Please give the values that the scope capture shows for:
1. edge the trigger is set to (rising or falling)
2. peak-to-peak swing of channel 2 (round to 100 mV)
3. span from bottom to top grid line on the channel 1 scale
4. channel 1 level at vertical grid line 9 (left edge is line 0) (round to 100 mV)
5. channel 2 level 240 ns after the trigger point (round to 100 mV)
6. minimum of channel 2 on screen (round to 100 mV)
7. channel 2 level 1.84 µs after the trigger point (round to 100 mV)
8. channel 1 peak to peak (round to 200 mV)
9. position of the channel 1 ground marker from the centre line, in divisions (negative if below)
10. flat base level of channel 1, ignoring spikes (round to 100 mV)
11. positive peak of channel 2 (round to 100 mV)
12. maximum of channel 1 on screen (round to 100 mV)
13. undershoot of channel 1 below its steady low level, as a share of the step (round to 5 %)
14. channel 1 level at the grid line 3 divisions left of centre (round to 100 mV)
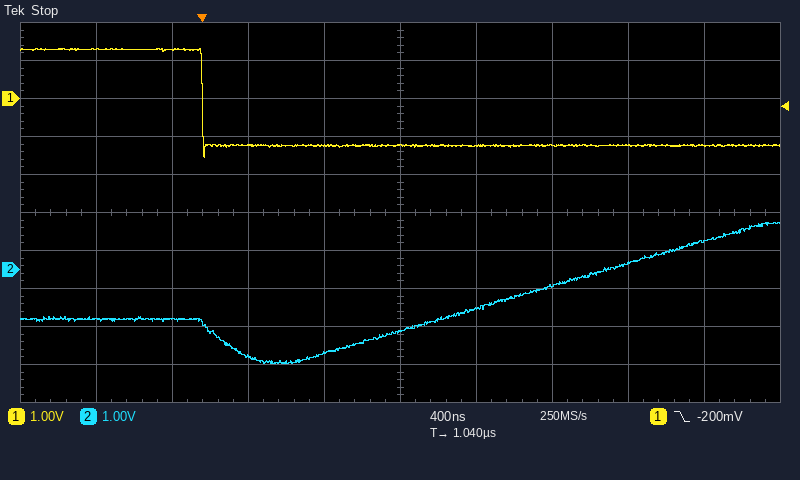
falling
3.7 V
10 V
-1.2 V
-2.3 V
-2.5 V
-400 mV
2.8 V
+3.0 div
-1.2 V
1.2 V
1.3 V
10 %
1.3 V
